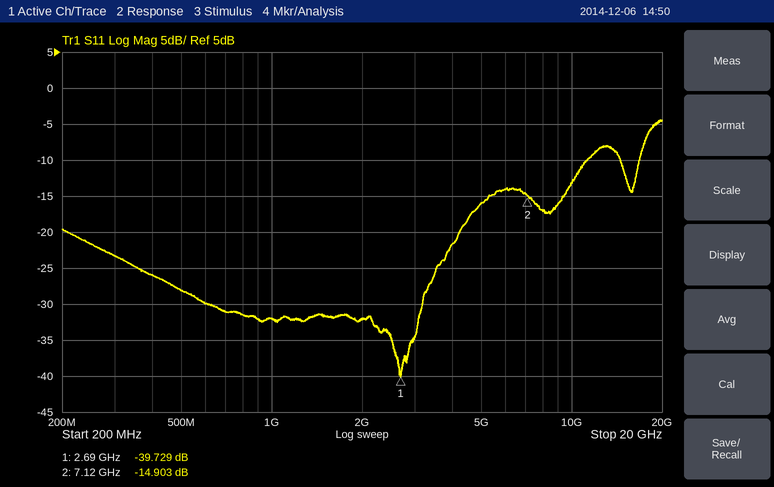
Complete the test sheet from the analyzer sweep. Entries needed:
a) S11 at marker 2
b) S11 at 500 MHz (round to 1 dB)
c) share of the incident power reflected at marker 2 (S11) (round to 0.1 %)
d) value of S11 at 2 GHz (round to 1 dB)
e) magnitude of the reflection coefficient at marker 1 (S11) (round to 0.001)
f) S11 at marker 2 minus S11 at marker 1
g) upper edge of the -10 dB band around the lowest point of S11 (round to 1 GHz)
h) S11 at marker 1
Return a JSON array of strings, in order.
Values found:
["-14.903 dB", "-28 dB", "3.2 %", "-32 dB", "0.010", "24.826 dB", "11 GHz", "-39.729 dB"]
